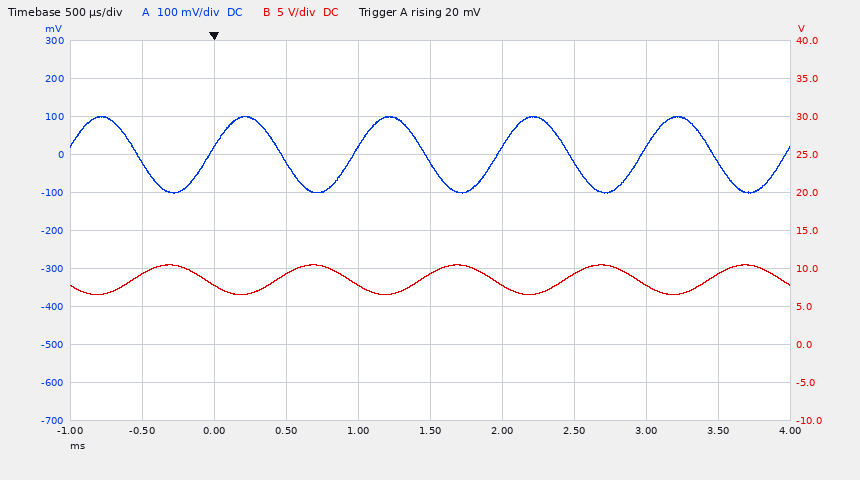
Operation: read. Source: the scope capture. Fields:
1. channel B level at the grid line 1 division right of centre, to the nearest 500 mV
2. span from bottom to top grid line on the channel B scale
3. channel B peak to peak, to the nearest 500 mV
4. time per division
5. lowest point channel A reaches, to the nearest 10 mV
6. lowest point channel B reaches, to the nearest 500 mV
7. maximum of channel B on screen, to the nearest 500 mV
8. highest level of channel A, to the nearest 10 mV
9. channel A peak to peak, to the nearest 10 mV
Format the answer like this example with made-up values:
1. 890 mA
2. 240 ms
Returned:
1. 8.0 V
2. 50 V
3. 4.0 V
4. 500 µs
5. -100 mV
6. 6.5 V
7. 10.5 V
8. 100 mV
9. 200 mV
